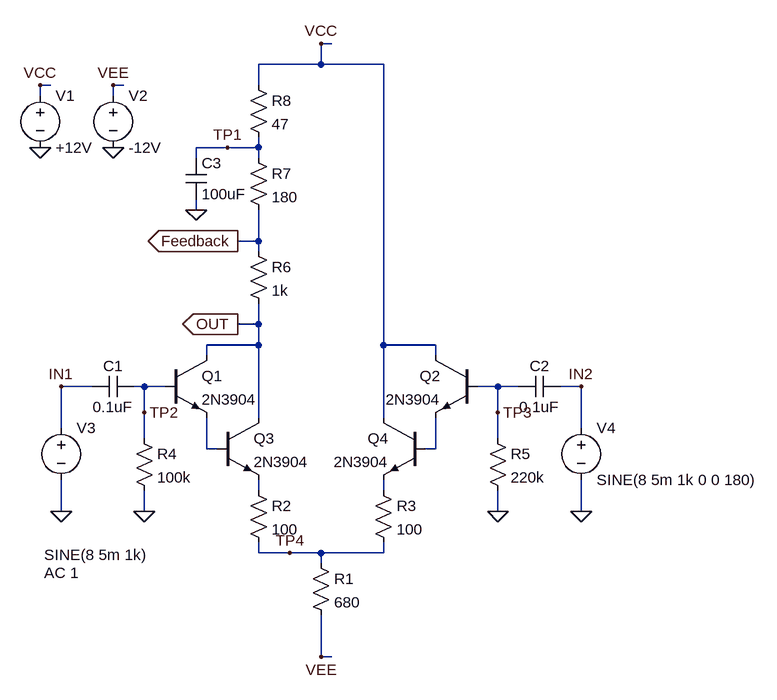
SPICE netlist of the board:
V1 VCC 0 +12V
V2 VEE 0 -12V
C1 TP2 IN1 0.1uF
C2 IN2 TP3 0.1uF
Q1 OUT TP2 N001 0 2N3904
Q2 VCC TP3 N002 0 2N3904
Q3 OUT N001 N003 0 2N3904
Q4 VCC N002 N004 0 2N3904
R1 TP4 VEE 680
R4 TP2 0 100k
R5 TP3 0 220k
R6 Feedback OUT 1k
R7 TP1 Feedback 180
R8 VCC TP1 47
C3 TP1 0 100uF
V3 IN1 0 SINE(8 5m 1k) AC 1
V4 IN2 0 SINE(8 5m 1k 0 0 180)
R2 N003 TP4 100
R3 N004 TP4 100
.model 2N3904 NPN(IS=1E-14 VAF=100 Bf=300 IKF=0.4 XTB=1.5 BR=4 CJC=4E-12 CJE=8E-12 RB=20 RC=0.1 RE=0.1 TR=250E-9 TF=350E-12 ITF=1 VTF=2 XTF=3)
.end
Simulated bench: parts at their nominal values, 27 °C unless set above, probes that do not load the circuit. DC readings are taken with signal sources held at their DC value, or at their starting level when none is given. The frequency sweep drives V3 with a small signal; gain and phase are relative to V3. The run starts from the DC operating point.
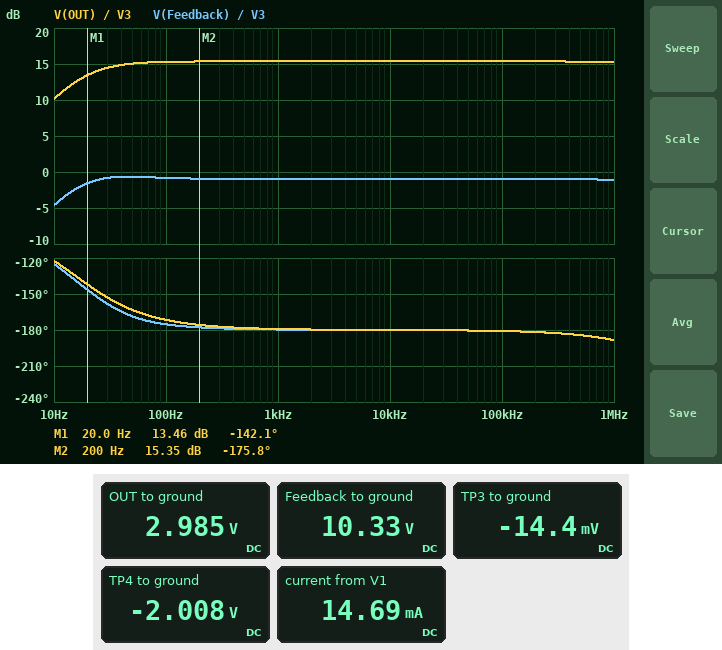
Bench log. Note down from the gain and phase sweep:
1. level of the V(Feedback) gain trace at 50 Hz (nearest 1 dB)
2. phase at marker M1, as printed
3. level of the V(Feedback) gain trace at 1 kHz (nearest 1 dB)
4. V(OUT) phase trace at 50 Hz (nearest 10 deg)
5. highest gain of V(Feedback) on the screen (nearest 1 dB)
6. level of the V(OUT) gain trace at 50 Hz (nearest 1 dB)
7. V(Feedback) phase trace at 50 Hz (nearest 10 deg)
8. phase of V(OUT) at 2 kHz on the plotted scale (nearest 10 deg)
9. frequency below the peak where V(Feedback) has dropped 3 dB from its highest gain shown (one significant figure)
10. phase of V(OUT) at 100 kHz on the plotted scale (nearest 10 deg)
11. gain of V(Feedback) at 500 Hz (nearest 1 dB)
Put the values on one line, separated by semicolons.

-1 dB; -142.1 deg; -1 dB; -160 deg; -1 dB; 15 dB; -170 deg; -180 deg; 10 Hz; -180 deg; -1 dB
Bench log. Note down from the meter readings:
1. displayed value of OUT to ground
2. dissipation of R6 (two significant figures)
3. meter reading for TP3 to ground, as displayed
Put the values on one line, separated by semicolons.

2.985 V; 54 mW; -14.4 mV
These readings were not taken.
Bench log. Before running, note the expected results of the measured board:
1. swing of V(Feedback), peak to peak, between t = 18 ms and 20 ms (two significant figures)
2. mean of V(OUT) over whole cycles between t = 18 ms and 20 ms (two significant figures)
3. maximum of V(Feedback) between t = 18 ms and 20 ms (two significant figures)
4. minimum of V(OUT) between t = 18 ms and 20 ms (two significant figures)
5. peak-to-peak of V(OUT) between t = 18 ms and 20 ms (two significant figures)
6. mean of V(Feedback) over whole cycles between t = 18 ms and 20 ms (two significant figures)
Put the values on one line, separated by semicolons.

17 mV; 3.0 V; 10 V; 2.9 V; 110 mV; 10 V
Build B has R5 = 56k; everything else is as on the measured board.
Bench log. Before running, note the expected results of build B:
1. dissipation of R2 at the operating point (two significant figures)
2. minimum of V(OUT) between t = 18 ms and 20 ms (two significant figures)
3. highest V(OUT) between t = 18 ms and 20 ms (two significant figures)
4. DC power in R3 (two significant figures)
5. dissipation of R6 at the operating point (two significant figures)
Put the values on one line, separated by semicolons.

5.3 mW; 3.0 V; 3.1 V; 5.5 mW; 53 mW
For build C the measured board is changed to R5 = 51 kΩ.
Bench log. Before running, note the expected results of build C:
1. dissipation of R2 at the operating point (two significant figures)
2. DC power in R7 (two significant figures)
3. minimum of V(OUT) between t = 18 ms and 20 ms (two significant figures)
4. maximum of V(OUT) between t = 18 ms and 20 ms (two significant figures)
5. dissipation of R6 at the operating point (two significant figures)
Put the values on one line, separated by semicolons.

5.3 mW; 9.6 mW; 3.0 V; 3.1 V; 53 mW
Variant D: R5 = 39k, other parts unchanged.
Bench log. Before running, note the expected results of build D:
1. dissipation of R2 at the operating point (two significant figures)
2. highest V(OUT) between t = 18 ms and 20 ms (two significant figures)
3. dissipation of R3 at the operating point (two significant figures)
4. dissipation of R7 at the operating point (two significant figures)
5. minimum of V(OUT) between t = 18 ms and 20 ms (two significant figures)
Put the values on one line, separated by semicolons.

5.3 mW; 3.1 V; 5.5 mW; 9.6 mW; 3.0 V
